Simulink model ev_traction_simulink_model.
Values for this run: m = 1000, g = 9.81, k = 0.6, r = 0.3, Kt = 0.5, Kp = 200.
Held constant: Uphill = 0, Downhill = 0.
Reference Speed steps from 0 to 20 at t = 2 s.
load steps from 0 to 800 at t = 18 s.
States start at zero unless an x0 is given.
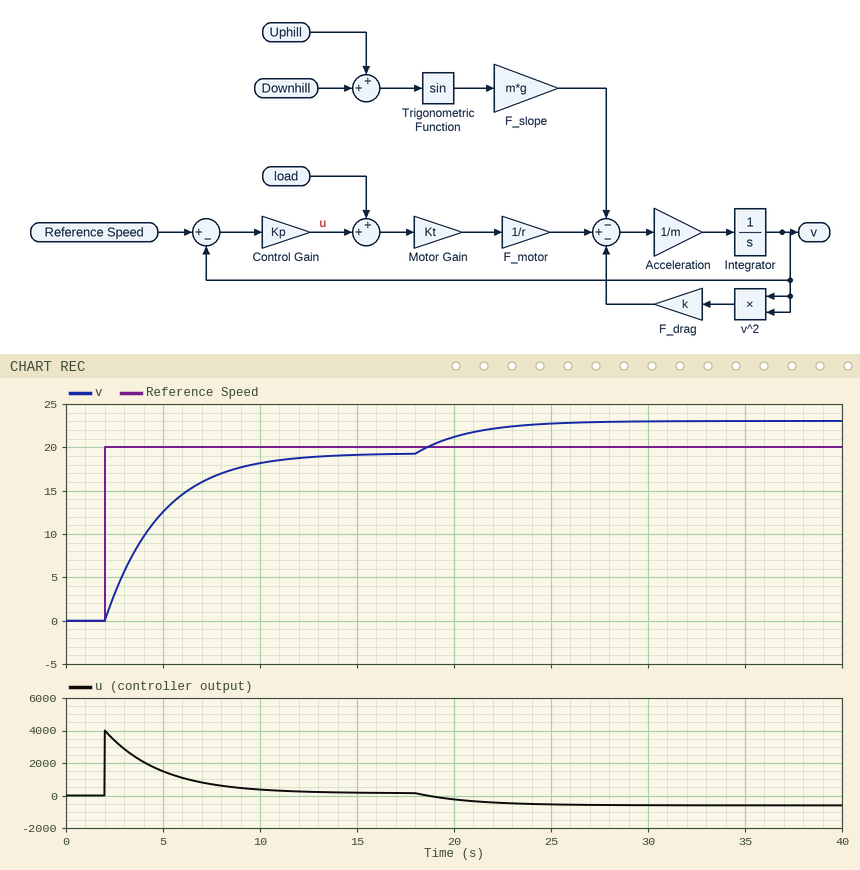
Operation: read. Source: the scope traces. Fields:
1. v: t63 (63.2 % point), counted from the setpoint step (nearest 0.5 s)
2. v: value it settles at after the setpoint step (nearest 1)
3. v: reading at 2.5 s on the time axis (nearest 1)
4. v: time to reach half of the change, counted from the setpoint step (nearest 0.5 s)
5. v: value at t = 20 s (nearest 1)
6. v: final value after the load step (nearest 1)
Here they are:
3.0 s
19
3
2.0 s
21
23
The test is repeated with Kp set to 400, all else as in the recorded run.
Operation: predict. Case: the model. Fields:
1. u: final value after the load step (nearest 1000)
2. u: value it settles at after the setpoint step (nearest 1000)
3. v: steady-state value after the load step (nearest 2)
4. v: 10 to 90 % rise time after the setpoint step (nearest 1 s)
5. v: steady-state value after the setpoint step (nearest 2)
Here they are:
-1000
0
22
3 s
20
